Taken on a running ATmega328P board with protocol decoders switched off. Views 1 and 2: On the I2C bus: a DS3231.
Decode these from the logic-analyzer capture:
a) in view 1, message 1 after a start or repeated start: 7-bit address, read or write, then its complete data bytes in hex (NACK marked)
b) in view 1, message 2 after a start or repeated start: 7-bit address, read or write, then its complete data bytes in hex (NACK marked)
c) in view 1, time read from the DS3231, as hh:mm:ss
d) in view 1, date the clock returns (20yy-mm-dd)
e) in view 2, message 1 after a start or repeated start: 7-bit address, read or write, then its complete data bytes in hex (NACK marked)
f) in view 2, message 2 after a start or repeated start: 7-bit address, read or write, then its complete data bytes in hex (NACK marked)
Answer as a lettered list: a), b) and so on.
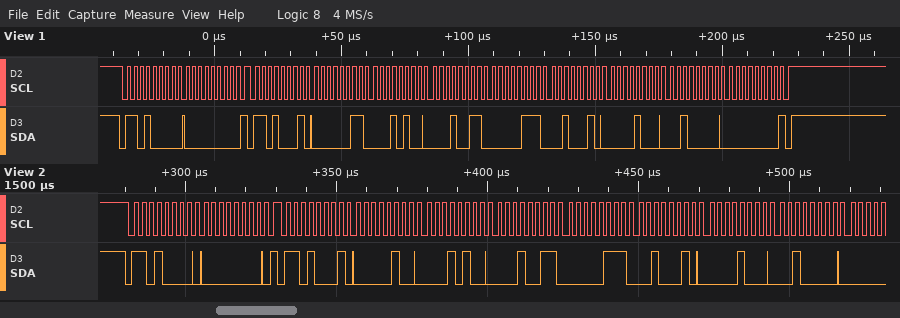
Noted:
a) 0x68 write: 00
b) 0x68 read: 03 14 13 07 22 08 20 00 NACK
c) 13:14:03
d) 2020-08-22
e) 0x68 write: 00
f) 0x68 read: 04 14 13 07 22 08 20
